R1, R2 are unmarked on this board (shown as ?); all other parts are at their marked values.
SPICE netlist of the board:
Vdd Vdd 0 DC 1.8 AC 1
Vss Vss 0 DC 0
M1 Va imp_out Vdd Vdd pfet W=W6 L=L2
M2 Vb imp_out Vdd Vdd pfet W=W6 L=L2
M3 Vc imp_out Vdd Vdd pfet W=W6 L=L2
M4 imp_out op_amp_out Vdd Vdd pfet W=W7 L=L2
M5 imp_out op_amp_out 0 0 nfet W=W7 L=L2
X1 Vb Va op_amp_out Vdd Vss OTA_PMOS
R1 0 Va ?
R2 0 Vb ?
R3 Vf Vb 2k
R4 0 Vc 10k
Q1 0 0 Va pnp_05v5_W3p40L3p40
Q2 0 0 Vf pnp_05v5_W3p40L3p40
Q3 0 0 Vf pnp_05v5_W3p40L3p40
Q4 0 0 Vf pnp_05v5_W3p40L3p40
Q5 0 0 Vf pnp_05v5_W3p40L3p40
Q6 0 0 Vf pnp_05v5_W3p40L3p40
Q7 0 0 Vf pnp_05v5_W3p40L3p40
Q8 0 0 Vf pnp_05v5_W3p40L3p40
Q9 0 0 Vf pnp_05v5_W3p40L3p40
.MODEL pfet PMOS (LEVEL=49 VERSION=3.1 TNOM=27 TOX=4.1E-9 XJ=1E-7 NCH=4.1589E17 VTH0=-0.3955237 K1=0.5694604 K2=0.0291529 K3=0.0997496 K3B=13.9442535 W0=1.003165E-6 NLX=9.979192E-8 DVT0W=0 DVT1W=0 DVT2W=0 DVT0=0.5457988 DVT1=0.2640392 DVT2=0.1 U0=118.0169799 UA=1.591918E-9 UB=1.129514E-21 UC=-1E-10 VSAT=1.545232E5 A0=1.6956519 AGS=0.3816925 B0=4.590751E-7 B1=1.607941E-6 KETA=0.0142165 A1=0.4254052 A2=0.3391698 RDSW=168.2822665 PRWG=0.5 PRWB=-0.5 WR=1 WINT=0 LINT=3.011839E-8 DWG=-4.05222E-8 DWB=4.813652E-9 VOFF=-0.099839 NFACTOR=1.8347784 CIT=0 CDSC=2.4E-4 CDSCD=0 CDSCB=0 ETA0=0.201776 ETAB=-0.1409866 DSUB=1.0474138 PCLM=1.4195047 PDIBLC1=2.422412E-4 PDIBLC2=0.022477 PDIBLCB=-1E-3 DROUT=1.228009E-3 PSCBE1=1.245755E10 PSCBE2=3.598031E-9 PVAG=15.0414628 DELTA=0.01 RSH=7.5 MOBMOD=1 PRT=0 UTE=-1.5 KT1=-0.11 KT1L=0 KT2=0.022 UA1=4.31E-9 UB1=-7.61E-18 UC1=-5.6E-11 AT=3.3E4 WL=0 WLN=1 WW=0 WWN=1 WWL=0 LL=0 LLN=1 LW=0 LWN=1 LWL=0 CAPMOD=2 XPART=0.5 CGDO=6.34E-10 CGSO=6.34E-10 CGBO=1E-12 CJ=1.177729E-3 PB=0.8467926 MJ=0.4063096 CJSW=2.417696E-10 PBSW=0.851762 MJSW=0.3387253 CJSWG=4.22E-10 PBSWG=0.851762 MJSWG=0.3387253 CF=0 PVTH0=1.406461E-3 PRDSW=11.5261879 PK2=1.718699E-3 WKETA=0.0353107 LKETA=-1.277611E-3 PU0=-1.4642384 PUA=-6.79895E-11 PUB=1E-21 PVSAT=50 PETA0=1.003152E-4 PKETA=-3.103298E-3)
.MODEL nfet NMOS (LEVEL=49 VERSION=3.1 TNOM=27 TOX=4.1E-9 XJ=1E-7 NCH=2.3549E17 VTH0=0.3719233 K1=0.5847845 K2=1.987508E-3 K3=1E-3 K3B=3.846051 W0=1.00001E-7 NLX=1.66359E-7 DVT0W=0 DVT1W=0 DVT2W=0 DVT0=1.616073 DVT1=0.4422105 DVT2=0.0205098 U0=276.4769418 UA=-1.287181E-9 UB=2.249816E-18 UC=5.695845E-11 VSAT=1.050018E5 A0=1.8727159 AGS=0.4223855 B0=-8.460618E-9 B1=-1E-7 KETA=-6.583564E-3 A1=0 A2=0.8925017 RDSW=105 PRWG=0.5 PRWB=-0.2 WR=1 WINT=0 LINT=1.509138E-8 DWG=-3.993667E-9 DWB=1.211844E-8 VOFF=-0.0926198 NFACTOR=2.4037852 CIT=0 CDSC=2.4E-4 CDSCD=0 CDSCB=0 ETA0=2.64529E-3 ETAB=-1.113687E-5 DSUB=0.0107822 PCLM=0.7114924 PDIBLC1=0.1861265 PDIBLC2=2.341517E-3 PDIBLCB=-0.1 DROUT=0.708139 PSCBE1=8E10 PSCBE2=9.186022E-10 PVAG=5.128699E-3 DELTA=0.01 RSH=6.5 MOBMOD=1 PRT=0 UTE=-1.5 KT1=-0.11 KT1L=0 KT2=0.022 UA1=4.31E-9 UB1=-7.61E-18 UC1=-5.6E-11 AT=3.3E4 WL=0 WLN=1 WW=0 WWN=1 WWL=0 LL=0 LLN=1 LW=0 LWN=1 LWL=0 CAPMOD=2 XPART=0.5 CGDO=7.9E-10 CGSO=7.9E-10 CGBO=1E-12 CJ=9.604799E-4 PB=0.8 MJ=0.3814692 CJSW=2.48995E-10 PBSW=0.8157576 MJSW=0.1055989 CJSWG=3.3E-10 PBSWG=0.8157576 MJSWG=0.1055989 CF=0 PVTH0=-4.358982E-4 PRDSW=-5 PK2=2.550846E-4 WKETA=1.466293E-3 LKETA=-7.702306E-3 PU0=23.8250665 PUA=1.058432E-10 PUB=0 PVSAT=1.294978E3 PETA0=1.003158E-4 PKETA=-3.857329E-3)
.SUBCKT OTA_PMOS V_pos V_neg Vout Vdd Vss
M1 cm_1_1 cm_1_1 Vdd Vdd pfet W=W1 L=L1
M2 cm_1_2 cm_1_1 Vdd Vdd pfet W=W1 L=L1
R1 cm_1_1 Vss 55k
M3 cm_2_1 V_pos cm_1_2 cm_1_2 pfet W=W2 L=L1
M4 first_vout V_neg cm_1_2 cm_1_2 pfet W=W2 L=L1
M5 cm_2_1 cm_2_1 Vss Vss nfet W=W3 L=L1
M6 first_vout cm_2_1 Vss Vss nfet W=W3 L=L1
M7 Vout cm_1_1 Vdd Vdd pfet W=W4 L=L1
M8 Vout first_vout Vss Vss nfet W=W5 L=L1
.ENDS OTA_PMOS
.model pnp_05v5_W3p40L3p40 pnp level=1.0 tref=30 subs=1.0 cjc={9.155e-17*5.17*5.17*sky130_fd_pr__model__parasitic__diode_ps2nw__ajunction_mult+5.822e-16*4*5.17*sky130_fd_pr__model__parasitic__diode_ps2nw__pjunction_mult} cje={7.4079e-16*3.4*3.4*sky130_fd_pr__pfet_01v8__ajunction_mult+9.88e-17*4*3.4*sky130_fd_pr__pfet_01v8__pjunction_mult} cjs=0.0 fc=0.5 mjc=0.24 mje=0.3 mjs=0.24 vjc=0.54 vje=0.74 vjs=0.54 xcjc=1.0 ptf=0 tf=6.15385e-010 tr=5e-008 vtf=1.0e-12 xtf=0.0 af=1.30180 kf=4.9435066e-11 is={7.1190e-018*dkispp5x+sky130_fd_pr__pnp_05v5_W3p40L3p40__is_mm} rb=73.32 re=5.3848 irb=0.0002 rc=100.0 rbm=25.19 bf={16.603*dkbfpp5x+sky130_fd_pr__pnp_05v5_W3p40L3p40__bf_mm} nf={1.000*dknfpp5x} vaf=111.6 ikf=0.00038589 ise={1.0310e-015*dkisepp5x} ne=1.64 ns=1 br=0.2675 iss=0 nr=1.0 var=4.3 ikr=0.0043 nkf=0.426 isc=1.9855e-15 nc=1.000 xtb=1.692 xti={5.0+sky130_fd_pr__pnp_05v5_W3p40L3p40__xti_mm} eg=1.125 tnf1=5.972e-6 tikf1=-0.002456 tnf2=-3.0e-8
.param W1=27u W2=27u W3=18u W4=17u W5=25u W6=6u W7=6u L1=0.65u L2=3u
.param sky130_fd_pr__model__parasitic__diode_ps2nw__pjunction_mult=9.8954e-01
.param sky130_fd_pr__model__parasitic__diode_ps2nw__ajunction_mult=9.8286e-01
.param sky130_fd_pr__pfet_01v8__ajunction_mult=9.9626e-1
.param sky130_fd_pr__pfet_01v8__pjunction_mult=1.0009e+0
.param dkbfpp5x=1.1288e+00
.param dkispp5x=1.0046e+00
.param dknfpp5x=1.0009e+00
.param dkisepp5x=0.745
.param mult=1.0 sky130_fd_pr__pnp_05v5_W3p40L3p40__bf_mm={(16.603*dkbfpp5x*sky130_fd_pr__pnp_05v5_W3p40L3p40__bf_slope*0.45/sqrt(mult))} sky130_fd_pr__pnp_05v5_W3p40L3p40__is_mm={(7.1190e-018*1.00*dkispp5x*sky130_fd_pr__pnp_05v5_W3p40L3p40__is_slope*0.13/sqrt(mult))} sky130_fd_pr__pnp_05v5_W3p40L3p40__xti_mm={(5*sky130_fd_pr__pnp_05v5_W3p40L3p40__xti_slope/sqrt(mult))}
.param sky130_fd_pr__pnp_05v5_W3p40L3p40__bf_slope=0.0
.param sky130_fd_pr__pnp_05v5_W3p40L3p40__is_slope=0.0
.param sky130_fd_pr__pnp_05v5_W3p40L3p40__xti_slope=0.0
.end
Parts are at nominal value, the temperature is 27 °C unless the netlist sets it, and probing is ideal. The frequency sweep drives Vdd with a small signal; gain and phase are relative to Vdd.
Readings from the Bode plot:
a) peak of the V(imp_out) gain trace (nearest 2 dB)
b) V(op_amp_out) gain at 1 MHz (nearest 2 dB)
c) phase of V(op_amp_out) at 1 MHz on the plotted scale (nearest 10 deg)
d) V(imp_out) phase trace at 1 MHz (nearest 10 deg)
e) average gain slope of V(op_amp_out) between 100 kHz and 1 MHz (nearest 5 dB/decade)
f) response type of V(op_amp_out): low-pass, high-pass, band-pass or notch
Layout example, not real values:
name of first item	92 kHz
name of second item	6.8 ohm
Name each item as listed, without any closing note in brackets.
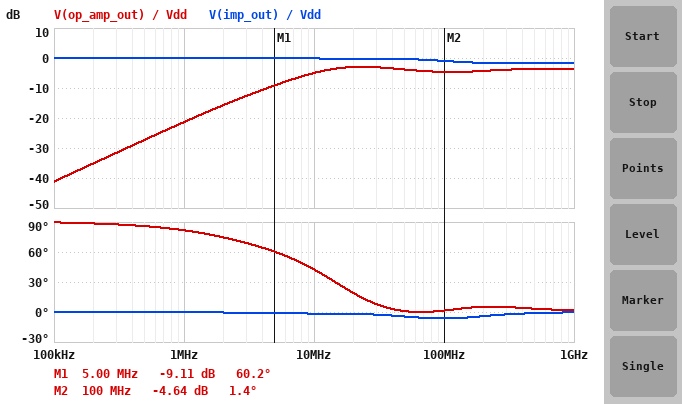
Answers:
peak of the V(imp_out) gain trace	0 dB
V(op_amp_out) gain at 1 MHz	-22 dB
phase of V(op_amp_out) at 1 MHz on the plotted scale	80 deg
V(imp_out) phase trace at 1 MHz	0 deg
average gain slope of V(op_amp_out) between 100 kHz and 1 MHz	20 dB/decade
response type of V(op_amp_out): low-pass, high-pass, band-pass or notch	high-pass
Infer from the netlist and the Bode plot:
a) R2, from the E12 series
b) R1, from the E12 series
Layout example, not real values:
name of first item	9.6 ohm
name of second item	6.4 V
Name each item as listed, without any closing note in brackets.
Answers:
R2, from the E12 series	56 kΩ
R1, from the E12 series	33 kΩ
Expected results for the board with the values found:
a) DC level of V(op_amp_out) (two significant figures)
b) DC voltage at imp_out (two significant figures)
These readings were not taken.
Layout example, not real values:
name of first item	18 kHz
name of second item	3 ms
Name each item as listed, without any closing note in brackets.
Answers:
DC level of V(op_amp_out)	200 mV
DC voltage at imp_out	1.8 V
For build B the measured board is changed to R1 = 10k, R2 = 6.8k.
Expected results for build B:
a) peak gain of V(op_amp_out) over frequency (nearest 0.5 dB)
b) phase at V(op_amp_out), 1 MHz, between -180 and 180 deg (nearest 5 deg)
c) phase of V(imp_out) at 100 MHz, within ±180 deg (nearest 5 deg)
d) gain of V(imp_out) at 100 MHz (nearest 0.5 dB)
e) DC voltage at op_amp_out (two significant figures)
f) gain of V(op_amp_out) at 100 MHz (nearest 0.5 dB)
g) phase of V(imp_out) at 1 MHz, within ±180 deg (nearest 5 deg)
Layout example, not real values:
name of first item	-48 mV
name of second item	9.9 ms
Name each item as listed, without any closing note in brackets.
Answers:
peak gain of V(op_amp_out) over frequency	0 dB
phase at V(op_amp_out), 1 MHz, between -180 and 180 deg	0 deg
phase of V(imp_out) at 100 MHz, within ±180 deg	65 deg
gain of V(imp_out) at 100 MHz	-8.5 dB
DC voltage at op_amp_out	1.8 V
gain of V(op_amp_out) at 100 MHz	-2.5 dB
phase of V(imp_out) at 1 MHz, within ±180 deg	90 deg
